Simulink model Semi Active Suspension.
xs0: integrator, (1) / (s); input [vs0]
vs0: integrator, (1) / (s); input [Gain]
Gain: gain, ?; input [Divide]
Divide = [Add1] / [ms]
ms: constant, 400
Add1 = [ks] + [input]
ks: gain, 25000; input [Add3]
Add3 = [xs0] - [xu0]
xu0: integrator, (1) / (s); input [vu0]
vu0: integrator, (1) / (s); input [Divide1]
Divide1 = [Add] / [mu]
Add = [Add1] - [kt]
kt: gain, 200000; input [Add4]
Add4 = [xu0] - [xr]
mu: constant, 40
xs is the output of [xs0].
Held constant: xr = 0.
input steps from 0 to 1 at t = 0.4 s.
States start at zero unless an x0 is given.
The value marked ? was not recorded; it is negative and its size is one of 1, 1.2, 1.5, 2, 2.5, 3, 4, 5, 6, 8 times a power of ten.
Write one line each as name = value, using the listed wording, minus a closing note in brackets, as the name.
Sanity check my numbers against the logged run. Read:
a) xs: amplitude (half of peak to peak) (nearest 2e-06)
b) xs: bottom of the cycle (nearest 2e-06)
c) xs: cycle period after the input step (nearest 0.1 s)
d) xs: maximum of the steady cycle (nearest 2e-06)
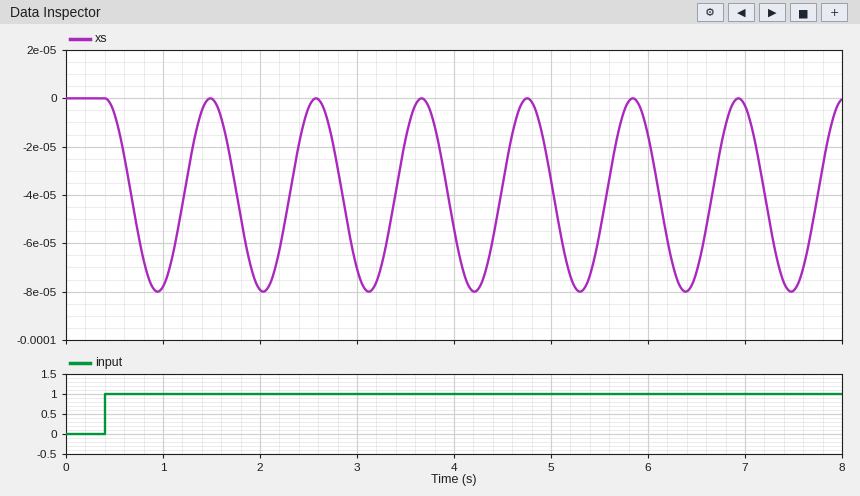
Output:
xs: amplitude (half of peak to peak) = 0.000040
xs: bottom of the cycle = -0.000080
xs: cycle period after the input step = 1.1 s
xs: maximum of the steady cycle = 0.000000
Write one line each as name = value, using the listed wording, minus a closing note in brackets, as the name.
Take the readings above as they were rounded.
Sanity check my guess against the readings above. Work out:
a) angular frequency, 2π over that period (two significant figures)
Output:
angular frequency, 2π over that period = 5.7 rad/s
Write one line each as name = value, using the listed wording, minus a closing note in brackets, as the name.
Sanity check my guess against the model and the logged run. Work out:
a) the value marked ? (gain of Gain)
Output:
the value marked ? = -0.6
